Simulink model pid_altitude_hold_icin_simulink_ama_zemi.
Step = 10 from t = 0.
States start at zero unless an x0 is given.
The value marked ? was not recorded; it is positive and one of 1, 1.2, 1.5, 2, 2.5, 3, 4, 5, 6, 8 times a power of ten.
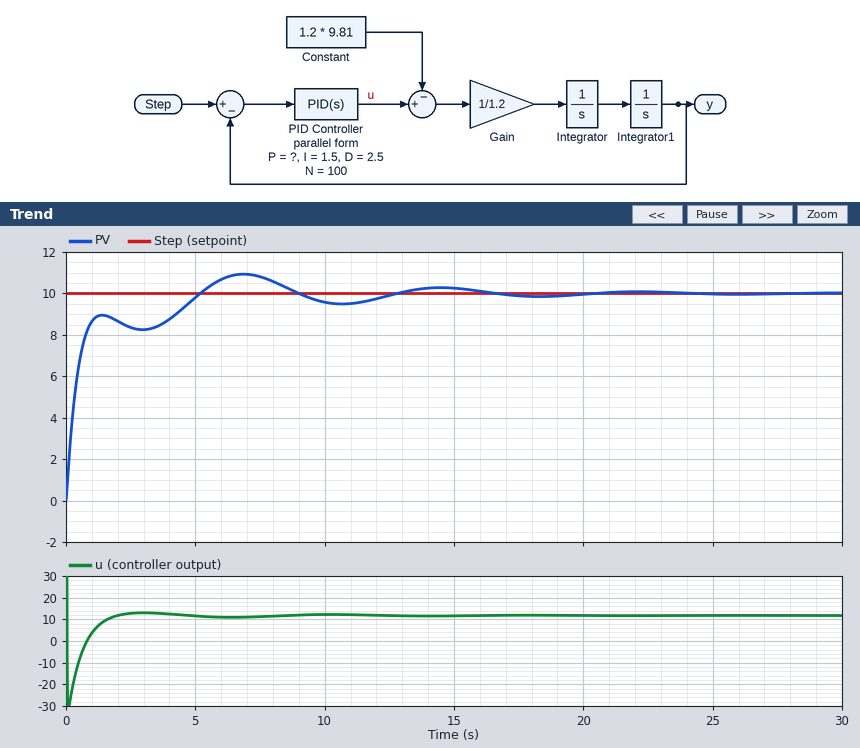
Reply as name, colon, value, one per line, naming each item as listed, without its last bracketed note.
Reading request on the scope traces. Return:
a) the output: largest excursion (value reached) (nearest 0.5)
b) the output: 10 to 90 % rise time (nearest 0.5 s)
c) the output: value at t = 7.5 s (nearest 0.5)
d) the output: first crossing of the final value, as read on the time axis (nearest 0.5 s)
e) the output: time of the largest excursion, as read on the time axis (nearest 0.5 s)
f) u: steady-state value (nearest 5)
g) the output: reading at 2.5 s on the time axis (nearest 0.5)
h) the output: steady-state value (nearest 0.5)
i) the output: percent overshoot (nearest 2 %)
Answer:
the output: largest excursion (value reached): 11.0
the output: 10 to 90 % rise time: 4.0 s
the output: value at t = 7.5 s: 11.0
the output: first crossing of the final value, as read on the time axis: 5.0 s
the output: time of the largest excursion, as read on the time axis: 7.0 s
u: steady-state value: 10
the output: reading at 2.5 s on the time axis: 8.5
the output: steady-state value: 10.0
the output: percent overshoot: 10 %
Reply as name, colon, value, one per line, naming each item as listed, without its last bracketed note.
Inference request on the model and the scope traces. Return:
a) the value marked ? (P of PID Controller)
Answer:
the value marked ?: 1.5
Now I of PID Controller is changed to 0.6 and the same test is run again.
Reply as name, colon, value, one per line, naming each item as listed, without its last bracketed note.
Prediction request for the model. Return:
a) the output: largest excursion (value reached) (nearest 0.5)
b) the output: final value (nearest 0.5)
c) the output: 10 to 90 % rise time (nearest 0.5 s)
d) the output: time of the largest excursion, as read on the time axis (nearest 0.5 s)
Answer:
the output: largest excursion (value reached): 10.5
the output: final value: 10.0
the output: 10 to 90 % rise time: 6.5 s
the output: time of the largest excursion, as read on the time axis: 10.0 s
